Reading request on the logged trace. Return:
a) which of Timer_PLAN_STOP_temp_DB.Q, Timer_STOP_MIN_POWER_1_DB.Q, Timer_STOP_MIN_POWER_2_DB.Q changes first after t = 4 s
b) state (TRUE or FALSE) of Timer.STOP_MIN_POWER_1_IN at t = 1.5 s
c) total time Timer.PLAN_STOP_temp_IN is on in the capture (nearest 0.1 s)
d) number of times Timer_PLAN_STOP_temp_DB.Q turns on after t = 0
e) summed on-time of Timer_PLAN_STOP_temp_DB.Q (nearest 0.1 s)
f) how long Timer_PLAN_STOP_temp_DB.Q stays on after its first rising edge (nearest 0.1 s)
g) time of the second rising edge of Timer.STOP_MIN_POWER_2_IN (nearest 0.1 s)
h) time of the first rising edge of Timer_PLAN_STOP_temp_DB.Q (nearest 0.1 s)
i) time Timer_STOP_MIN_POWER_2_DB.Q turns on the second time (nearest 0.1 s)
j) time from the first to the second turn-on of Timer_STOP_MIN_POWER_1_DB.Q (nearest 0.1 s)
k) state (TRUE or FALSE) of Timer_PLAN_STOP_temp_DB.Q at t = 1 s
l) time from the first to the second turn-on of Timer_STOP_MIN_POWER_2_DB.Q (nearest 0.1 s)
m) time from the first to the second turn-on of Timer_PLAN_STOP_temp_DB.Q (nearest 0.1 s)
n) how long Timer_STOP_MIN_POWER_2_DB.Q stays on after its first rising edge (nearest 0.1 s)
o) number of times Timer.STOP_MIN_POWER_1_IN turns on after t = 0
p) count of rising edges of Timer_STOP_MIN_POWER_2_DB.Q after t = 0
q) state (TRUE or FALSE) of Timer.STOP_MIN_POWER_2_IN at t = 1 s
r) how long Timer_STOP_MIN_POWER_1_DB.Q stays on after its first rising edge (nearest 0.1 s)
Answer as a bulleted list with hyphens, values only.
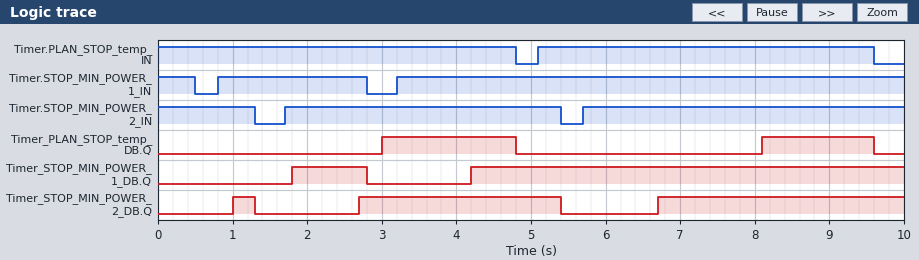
- Timer_STOP_MIN_POWER_1_DB.Q
- TRUE
- 9.3 s
- 2
- 3.3 s
- 1.8 s
- 5.7 s
- 3.0 s
- 2.7 s
- 2.4 s
- FALSE
- 1.7 s
- 5.1 s
- 0.3 s
- 2
- 3
- TRUE
- 1.0 s
